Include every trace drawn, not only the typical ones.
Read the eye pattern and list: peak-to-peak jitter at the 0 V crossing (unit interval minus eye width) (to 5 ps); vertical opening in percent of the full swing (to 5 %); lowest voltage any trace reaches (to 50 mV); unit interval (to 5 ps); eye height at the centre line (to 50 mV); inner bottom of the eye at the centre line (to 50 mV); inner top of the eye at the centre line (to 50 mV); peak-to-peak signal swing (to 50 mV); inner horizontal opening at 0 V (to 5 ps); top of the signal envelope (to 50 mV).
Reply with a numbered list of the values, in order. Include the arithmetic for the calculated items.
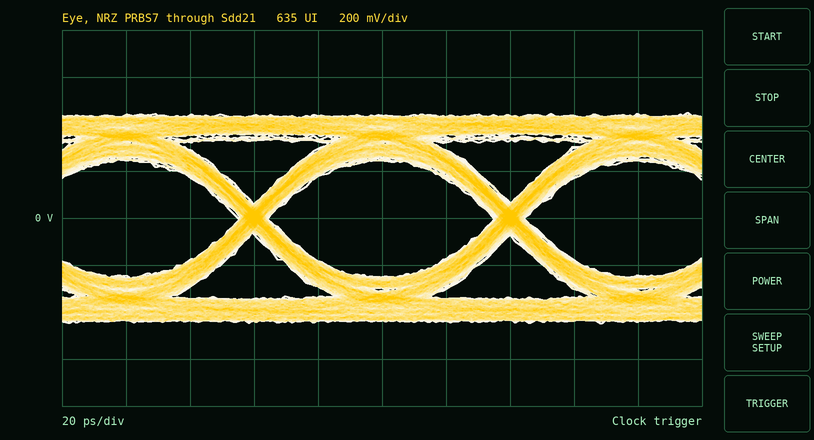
1. 10 ps
2. 500 mV / 900 mV ≈ 55.6 %, so 55 % to the nearest 5 %
3. -450 mV
4. 80 ps
5. 500 mV
6. -250 mV
7. 250 mV
8. 900 mV
9. 70 ps
10. 450 mV
